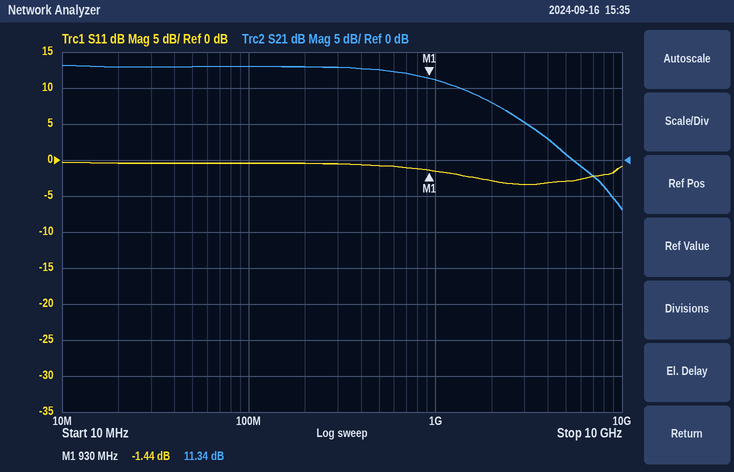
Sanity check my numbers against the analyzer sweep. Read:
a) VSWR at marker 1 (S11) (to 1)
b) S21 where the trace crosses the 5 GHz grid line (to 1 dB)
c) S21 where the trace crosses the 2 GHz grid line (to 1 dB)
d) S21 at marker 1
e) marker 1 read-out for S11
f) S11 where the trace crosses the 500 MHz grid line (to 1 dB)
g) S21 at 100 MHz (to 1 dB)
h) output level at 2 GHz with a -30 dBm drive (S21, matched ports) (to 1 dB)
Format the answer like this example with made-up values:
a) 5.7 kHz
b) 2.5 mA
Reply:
a) 12
b) 1 dB
c) 8 dB
d) 11.34 dB
e) -1.44 dB
f) -1 dB
g) 13 dB
h) -22 dBm
